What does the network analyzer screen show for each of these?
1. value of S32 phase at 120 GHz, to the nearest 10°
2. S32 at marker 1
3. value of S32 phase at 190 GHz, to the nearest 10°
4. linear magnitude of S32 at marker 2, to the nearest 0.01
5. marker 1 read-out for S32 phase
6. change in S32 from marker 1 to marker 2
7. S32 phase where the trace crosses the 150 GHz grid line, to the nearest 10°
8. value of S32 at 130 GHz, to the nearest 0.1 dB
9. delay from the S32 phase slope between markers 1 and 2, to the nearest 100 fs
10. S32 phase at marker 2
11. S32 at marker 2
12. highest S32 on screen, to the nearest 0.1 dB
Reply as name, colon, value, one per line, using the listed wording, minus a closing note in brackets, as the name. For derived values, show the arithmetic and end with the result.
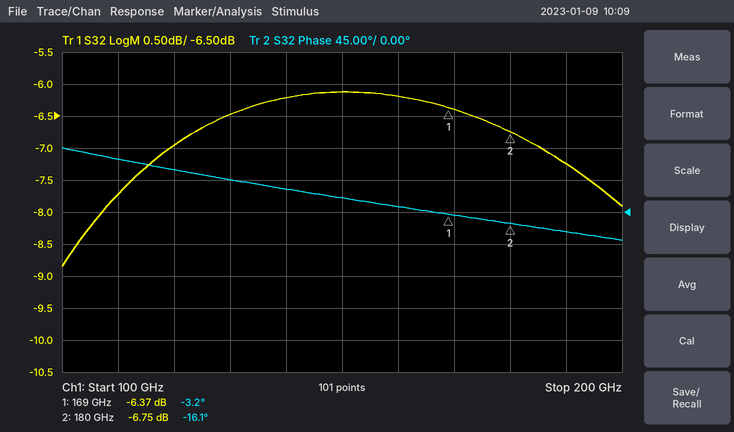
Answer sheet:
value of S32 phase at 120 GHz, to the nearest 10°: 60°
S32 at marker 1: -6.37 dB
value of S32 phase at 190 GHz, to the nearest 10°: -30°
linear magnitude of S32 at marker 2, to the nearest 0.01: 10^(-6.75/20) ≈ 0.46
marker 1 read-out for S32 phase: -3.2°
change in S32 from marker 1 to marker 2: -6.75 − (-6.37) = -0.38 dB
S32 phase where the trace crosses the 150 GHz grid line, to the nearest 10°: 20°
value of S32 at 130 GHz, to the nearest 0.1 dB: -6.5 dB
delay from the S32 phase slope between markers 1 and 2, to the nearest 100 fs: −(-16.1° − (-3.2°))/(360° × 11 GHz) ≈ 3.3 ps
S32 phase at marker 2: -16.1°
S32 at marker 2: -6.75 dB
highest S32 on screen, to the nearest 0.1 dB: -6.1 dB
